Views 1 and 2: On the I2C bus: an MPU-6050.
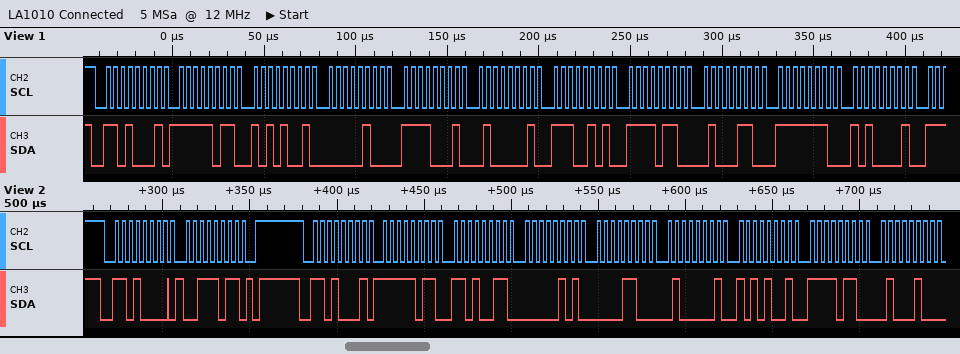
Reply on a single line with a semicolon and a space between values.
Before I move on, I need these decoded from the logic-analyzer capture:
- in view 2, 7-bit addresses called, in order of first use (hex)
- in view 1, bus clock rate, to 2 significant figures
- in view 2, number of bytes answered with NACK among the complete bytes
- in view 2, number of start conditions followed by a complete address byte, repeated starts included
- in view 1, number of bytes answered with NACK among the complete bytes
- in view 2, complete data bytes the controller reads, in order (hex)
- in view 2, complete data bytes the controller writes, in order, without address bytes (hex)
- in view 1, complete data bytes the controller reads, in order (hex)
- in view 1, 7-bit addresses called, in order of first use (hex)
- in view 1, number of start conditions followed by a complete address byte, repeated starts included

0x68; 250 kHz; 0; 2; 0; FB D3 05 0C 41 A9 F6 44; 3B; FB A9 04 F1 41 E5 F6 46 FE A1; 0x68; 1
